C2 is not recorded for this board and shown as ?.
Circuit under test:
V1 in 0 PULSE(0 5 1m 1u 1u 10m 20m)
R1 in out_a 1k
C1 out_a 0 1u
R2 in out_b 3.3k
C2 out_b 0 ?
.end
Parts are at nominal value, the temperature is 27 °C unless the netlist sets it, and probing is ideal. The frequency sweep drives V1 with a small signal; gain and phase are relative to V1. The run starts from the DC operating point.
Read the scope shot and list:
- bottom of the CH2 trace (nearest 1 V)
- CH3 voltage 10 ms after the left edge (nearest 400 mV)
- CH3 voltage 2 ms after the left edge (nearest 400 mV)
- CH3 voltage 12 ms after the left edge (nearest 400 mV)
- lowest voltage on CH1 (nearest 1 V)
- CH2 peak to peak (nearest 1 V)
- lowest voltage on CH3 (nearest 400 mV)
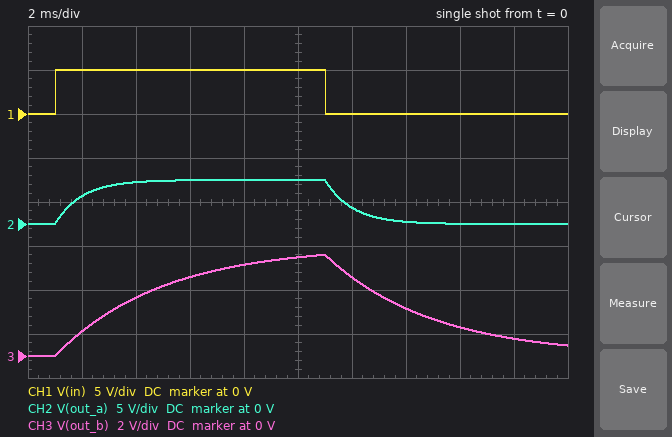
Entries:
0 V
4.4 V
1.2 V
3.6 V
0 V
5 V
0 V
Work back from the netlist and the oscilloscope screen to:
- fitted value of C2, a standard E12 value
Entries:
1.2 µF
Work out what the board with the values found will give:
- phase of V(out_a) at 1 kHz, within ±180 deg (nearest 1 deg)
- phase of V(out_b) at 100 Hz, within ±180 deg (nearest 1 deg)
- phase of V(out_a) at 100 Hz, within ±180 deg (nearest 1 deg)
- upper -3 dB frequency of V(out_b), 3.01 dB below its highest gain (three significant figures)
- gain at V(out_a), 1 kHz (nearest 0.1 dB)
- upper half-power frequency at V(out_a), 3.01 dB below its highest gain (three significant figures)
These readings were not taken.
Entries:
-81 deg
-68 deg
-32 deg
40.2 Hz
-16.1 dB
159 Hz
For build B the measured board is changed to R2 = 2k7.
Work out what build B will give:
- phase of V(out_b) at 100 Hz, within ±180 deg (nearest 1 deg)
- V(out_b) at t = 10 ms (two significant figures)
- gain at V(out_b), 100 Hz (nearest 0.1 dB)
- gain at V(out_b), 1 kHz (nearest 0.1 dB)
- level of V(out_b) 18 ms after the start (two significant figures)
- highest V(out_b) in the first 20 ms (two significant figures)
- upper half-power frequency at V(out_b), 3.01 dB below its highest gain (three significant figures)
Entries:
-64 deg
4.7 V
-7.1 dB
-26.2 dB
550 mV
4.8 V
49.1 Hz
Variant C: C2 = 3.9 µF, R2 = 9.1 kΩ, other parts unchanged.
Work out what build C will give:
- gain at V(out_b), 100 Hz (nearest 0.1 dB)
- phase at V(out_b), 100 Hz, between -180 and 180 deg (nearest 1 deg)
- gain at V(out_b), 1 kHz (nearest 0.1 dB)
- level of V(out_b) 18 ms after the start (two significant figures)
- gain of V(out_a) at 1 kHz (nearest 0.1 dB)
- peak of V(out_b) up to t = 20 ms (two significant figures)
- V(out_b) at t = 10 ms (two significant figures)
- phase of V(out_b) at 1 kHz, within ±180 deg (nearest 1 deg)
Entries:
-27.0 dB
-87 deg
-47.0 dB
1.0 V
-16.1 dB
1.2 V
1.1 V
-90 deg
